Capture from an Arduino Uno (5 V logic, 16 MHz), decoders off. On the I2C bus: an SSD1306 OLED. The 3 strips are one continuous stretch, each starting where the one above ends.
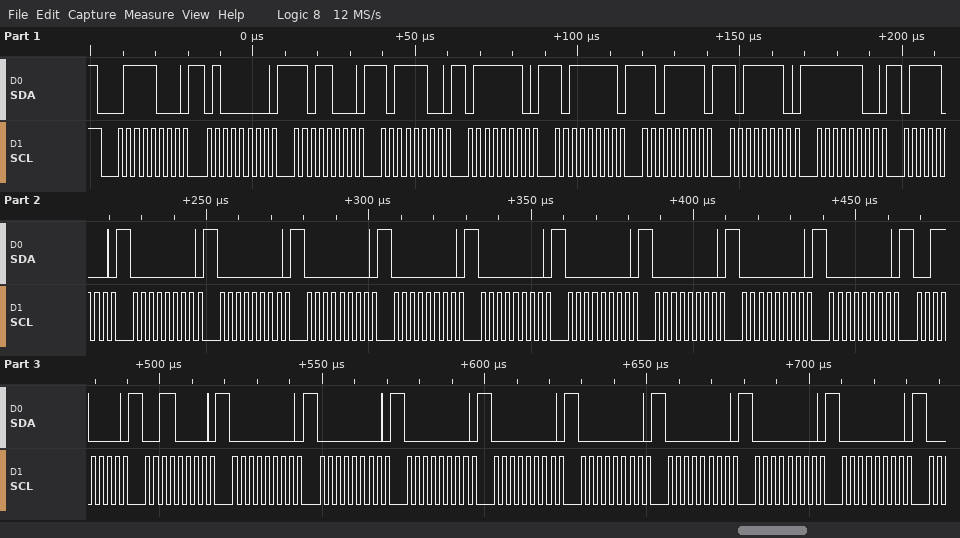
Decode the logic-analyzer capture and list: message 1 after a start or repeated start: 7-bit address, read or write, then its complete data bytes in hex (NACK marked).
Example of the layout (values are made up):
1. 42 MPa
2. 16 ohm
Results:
1. 0x3C write: 40 D8 BC 7E BF DF BE FC 78 00 00 00 00 00 00 00 00 00 30 30 00 00 00 00 00 00 00 00
